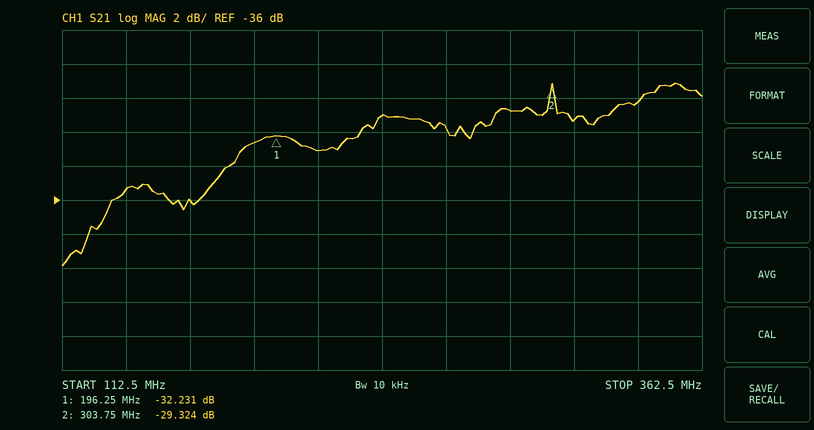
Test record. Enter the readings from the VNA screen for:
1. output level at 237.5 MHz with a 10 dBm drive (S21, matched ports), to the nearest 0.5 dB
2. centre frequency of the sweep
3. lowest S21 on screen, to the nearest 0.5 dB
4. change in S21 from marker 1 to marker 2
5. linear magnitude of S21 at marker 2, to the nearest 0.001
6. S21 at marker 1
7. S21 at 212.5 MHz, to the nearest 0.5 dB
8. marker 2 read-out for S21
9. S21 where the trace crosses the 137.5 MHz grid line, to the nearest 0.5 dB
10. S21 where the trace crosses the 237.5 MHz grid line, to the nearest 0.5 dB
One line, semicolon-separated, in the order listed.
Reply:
-21.0 dBm; 237.5 MHz; -40.0 dB; 2.907 dB; 0.034; -32.231 dB; -33.0 dB; -29.324 dB; -35.5 dB; -31.0 dB
